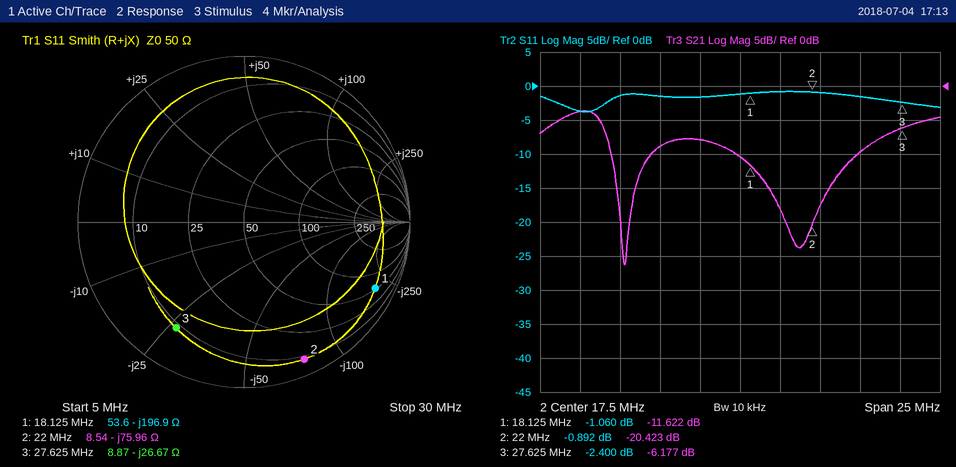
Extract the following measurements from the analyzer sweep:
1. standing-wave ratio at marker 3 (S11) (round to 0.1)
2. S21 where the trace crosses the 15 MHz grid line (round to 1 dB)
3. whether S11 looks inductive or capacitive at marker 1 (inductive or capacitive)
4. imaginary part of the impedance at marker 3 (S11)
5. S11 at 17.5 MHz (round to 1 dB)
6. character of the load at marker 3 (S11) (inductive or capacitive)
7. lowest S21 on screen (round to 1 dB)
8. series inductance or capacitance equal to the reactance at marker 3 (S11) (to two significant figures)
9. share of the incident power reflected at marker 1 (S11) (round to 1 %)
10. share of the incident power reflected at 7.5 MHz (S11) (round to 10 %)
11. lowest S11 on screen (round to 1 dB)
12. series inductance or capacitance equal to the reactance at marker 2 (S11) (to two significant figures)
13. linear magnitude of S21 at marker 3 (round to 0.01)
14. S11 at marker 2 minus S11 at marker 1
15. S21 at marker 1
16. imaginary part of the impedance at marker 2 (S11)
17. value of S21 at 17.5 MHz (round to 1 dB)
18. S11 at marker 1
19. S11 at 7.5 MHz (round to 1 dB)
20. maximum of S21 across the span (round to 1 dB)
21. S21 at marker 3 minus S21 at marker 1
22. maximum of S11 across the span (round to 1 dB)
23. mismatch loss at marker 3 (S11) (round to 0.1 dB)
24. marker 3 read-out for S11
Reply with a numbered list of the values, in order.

1. 7.3
2. -8 dB
3. capacitive
4. -26.67 Ω
5. -1 dB
6. capacitive
7. -26 dB
8. 220 pF
9. 78 %
10. 40 %
11. -4 dB
12. 95 pF
13. 0.49
14. 0.168 dB
15. -11.622 dB
16. -75.96 Ω
17. -10 dB
18. -1.060 dB
19. -4 dB
20. -4 dB
21. 5.445 dB
22. -1 dB
23. 3.7 dB
24. -2.400 dB
